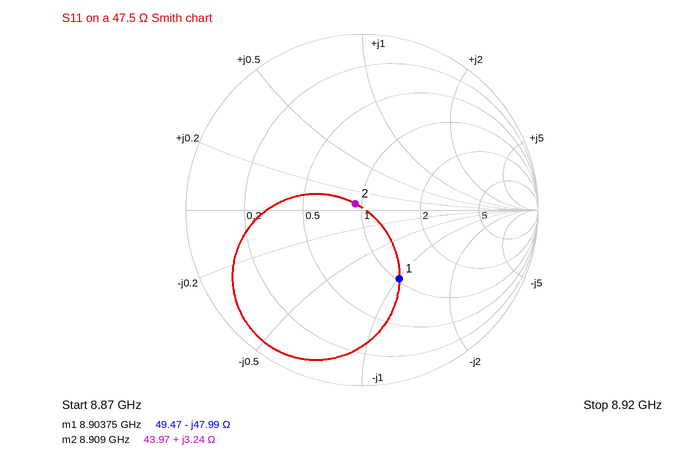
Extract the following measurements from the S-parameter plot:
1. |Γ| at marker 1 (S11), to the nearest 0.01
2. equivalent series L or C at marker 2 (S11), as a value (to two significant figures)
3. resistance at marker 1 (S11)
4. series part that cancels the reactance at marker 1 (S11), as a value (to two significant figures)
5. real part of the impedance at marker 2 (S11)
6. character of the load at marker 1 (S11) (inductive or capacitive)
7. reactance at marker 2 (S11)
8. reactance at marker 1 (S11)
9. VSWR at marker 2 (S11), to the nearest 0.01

0.44
58 pH
49.47 Ω
860 pH
43.97 Ω
capacitive
+3.24 Ω
-47.99 Ω
1.11
